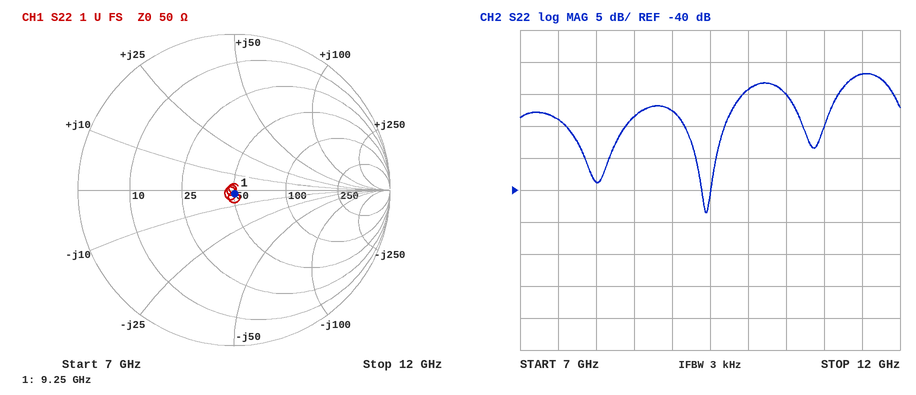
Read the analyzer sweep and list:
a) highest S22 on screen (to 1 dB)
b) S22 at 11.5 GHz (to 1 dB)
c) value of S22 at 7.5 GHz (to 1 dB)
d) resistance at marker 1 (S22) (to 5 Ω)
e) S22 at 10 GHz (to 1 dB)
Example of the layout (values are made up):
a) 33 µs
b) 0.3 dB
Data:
a) -22 dB
b) -22 dB
c) -29 dB
d) 50 Ω
e) -24 dB
